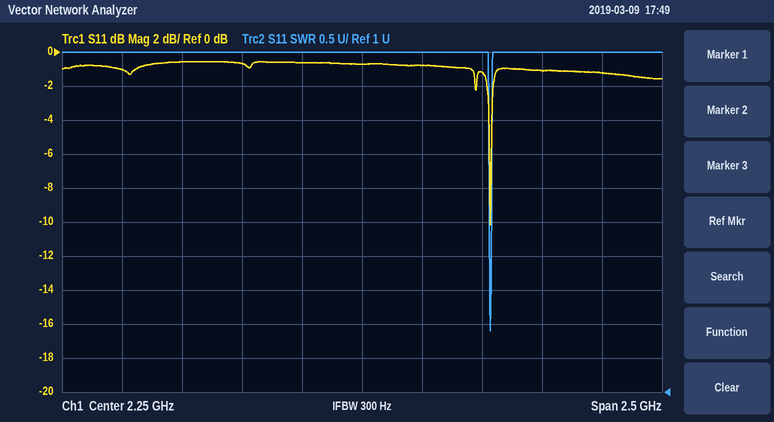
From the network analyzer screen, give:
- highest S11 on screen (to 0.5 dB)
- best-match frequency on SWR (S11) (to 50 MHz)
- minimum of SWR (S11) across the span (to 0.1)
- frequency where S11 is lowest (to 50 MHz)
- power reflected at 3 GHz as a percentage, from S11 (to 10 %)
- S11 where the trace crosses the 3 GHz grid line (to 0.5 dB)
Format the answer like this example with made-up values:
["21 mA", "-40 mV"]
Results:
["-0.5 dB", "2.80 GHz", "1.9", "2.80 GHz", "80 %", "-1.0 dB"]
